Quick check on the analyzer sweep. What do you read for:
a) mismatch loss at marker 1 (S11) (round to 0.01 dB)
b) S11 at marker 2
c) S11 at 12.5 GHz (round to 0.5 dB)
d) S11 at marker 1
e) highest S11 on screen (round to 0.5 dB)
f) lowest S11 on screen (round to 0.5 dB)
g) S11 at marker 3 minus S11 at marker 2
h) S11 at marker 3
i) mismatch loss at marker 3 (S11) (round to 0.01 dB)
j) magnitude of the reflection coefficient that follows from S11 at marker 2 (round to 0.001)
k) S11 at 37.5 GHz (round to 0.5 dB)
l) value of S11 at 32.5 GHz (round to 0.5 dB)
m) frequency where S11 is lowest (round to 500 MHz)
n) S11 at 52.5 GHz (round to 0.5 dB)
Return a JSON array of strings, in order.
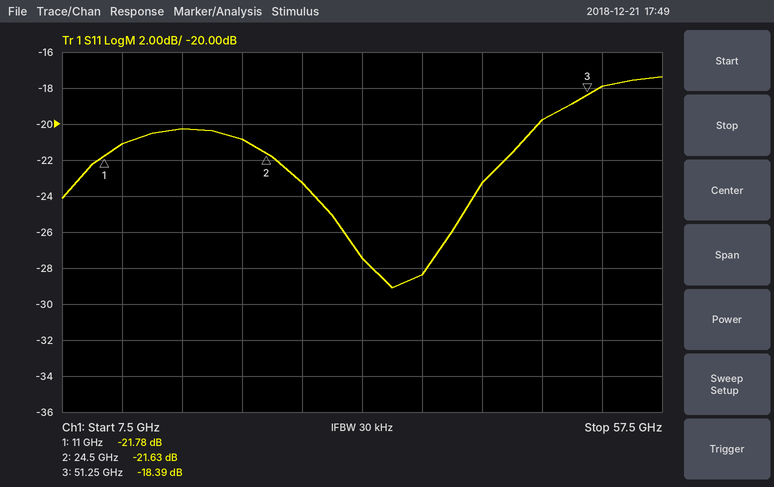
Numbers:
["0.03 dB", "-21.63 dB", "-21.0 dB", "-21.78 dB", "-17.5 dB", "-29.0 dB", "3.24 dB", "-18.39 dB", "0.06 dB", "0.083", "-28.5 dB", "-27.5 dB", "35.0 GHz", "-18.0 dB"]
